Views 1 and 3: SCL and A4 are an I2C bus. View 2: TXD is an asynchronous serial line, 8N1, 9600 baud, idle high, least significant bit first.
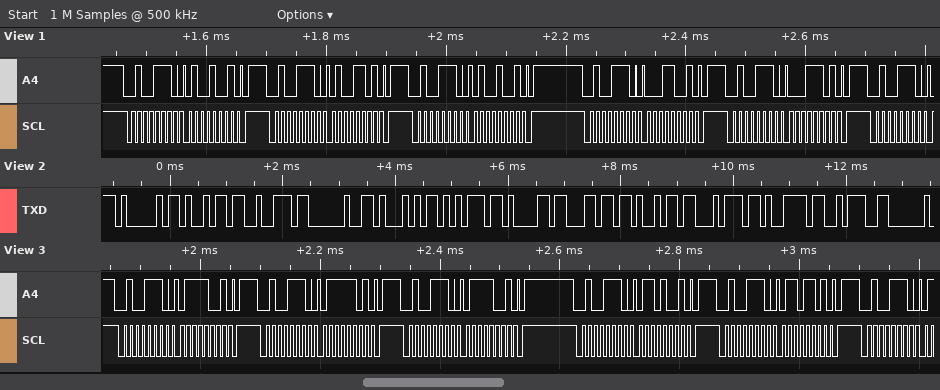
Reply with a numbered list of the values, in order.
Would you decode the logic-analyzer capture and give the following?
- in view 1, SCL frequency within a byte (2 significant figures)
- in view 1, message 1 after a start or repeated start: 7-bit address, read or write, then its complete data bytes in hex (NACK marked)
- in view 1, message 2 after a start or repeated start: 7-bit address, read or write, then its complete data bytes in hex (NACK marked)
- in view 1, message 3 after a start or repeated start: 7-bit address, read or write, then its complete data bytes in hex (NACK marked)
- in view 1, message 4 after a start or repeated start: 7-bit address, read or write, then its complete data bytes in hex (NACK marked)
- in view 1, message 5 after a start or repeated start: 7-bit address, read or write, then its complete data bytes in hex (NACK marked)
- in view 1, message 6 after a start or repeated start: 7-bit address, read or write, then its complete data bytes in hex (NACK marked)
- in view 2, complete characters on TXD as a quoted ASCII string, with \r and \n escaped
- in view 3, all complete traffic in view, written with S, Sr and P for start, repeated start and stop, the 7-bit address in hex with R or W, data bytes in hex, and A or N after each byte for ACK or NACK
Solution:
1. 100 kHz
2. 0x27 write: 49
3. 0x27 write: 4D
4. 0x27 write: 49
5. 0x27 write: 19
6. 0x27 write: 1D
7. 0x27 write
8. "Air Quality:"
9. S 27W A 79 A P S 27W A 7D A P S 27W A 79 A P S 27W A 69 A P S 27W A 6D A P S 27W A
